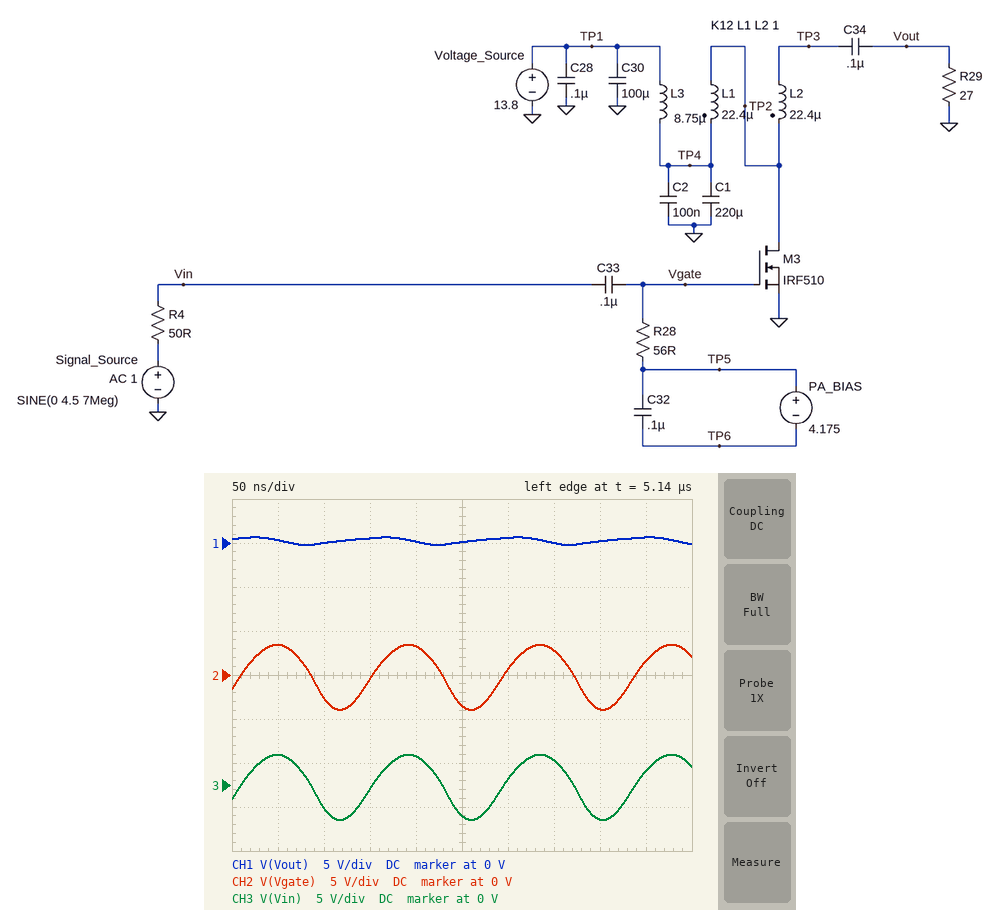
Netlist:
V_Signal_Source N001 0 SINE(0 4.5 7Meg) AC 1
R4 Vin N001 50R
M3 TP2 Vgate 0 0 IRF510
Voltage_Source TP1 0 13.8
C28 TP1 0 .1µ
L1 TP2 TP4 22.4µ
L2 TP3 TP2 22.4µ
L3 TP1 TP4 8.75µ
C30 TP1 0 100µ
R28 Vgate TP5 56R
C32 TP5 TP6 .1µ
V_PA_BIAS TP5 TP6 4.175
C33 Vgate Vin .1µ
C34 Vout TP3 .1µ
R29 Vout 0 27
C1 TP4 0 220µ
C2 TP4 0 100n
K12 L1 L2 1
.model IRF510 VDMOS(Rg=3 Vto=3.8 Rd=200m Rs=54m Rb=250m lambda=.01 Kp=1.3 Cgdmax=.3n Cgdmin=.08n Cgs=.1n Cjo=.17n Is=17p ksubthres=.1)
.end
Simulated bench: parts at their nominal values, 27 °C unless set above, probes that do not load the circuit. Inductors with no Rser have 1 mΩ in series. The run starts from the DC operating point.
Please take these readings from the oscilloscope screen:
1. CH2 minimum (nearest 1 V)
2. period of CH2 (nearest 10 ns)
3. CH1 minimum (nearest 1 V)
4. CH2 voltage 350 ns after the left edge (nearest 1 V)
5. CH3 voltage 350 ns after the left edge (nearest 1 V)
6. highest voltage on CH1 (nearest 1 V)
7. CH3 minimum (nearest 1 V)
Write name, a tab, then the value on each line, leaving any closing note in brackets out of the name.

CH2 minimum	-4 V
period of CH2	140 ns
CH1 minimum	0 V
CH2 voltage 350 ns after the left edge	3 V
CH3 voltage 350 ns after the left edge	3 V
highest voltage on CH1	1 V
CH3 minimum	-4 V
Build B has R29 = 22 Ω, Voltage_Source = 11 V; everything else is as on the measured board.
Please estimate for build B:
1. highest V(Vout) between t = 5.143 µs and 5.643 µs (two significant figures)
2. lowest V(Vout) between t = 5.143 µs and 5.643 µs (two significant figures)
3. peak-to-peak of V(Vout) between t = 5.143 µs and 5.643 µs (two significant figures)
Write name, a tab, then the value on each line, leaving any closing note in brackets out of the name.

highest V(Vout) between t = 5.143 µs and 5.643 µs	500 mV
lowest V(Vout) between t = 5.143 µs and 5.643 µs	-250 mV
peak-to-peak of V(Vout) between t = 5.143 µs and 5.643 µs	750 mV
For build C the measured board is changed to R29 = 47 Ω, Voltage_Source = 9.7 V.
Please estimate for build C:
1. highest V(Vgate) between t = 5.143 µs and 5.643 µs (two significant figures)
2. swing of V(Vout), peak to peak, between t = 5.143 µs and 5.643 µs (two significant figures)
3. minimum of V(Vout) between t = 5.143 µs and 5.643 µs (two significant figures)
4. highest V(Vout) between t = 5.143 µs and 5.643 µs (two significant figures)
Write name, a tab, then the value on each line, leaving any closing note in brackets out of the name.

highest V(Vgate) between t = 5.143 µs and 5.643 µs	3.4 V
swing of V(Vout), peak to peak, between t = 5.143 µs and 5.643 µs	1.6 V
minimum of V(Vout) between t = 5.143 µs and 5.643 µs	-620 mV
highest V(Vout) between t = 5.143 µs and 5.643 µs	940 mV
